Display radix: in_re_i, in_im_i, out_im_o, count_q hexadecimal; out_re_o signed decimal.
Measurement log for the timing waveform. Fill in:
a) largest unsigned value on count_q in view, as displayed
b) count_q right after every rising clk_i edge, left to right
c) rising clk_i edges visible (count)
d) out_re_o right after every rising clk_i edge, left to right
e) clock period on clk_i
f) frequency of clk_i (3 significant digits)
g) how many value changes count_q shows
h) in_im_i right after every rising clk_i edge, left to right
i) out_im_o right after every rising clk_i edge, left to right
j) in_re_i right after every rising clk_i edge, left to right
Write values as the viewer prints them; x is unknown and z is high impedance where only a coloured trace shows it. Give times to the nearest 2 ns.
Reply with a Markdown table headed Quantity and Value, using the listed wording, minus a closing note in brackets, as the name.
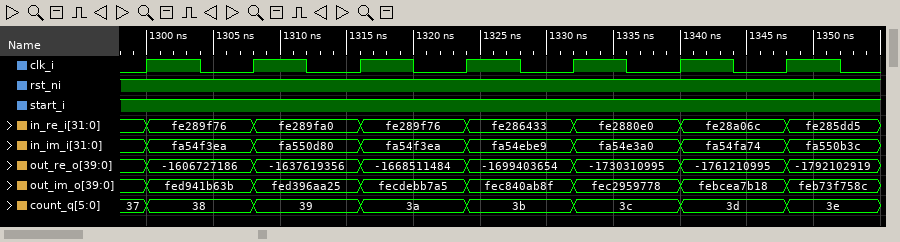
| Quantity | Value |
|---|---|
| largest unsigned value on count_q in view, as displayed | 3e |
| count_q right after every rising clk_i edge, left to right | 38, 39, 3a, 3b, 3c, 3d, 3e |
| rising clk_i edges visible | 7 |
| out_re_o right after every rising clk_i edge, left to right | -1606727186, -1637619356, -1668511484, -1699403654, -1730310995, -1761210995, -1792102919 |
| clock period on clk_i | 8 ns |
| frequency of clk_i | 125 MHz |
| how many value changes count_q shows | 7 |
| in_im_i right after every rising clk_i edge, left to right | fa54f3ea, fa550d80, fa54f3ea, fa54ebe9, fa54e3a0, fa54fa74, fa550b3c |
| out_im_o right after every rising clk_i edge, left to right | fed941b63b, fed396aa25, fecdebb7a5, fec840ab8f, fec2959778, febcea7b18, feb73f758c |
| in_re_i right after every rising clk_i edge, left to right | fe289f76, fe289fa0, fe289f76, fe286433, fe2880e0, fe28a06c, fe285dd5 |
